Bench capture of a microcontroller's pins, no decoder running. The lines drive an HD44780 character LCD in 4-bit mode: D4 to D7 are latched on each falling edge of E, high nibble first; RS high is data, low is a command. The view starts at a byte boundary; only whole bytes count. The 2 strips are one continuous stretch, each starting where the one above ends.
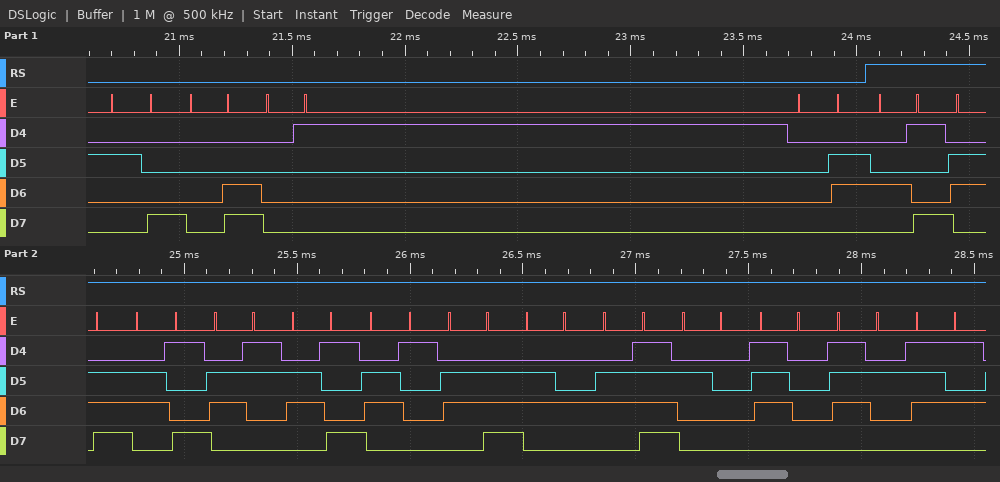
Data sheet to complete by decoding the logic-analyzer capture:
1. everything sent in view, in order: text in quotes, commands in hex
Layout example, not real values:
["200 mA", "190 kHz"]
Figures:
["0x28 0x0C 0x01 0x06 \"Iniciando pru\""]
